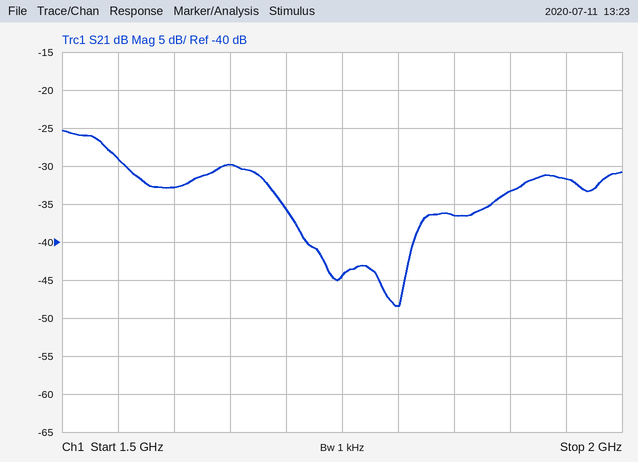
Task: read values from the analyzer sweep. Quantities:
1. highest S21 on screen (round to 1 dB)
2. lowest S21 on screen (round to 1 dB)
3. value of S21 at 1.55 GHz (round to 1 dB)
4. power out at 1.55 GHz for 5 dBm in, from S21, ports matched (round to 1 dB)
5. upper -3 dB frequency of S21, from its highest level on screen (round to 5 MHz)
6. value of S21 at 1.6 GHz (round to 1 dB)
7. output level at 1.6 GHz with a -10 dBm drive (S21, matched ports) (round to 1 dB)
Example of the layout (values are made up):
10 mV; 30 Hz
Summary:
-25 dB; -48 dB; -29 dB; -24 dBm; 1.545 GHz; -33 dB; -43 dBm
